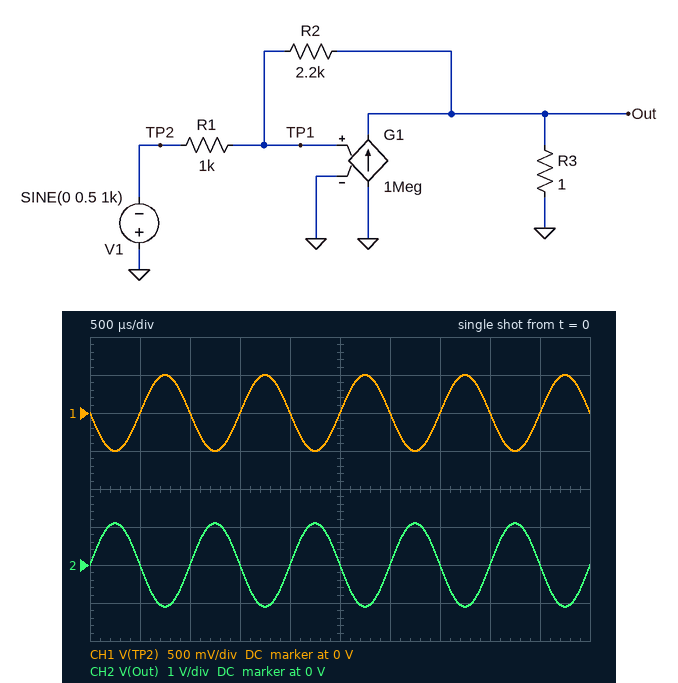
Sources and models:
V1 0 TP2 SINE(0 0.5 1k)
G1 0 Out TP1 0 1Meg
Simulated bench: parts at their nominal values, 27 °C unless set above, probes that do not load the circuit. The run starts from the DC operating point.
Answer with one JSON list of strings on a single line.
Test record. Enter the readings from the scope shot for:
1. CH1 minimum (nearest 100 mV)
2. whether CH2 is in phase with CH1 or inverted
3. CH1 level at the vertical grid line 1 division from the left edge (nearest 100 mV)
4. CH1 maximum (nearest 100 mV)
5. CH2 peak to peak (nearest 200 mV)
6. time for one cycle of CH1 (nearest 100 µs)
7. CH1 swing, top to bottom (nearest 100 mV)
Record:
["-500 mV", "inverted", "0 V", "500 mV", "2.2 V", "1.0 ms", "1.0 V"]
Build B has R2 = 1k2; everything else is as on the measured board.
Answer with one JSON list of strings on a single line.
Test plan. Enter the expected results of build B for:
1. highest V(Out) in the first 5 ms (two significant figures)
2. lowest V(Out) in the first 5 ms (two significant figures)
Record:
["600 mV", "-600 mV"]
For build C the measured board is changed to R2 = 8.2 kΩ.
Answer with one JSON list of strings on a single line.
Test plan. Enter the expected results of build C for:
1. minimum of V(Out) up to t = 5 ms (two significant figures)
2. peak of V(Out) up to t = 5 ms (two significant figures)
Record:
["-4.1 V", "4.1 V"]
